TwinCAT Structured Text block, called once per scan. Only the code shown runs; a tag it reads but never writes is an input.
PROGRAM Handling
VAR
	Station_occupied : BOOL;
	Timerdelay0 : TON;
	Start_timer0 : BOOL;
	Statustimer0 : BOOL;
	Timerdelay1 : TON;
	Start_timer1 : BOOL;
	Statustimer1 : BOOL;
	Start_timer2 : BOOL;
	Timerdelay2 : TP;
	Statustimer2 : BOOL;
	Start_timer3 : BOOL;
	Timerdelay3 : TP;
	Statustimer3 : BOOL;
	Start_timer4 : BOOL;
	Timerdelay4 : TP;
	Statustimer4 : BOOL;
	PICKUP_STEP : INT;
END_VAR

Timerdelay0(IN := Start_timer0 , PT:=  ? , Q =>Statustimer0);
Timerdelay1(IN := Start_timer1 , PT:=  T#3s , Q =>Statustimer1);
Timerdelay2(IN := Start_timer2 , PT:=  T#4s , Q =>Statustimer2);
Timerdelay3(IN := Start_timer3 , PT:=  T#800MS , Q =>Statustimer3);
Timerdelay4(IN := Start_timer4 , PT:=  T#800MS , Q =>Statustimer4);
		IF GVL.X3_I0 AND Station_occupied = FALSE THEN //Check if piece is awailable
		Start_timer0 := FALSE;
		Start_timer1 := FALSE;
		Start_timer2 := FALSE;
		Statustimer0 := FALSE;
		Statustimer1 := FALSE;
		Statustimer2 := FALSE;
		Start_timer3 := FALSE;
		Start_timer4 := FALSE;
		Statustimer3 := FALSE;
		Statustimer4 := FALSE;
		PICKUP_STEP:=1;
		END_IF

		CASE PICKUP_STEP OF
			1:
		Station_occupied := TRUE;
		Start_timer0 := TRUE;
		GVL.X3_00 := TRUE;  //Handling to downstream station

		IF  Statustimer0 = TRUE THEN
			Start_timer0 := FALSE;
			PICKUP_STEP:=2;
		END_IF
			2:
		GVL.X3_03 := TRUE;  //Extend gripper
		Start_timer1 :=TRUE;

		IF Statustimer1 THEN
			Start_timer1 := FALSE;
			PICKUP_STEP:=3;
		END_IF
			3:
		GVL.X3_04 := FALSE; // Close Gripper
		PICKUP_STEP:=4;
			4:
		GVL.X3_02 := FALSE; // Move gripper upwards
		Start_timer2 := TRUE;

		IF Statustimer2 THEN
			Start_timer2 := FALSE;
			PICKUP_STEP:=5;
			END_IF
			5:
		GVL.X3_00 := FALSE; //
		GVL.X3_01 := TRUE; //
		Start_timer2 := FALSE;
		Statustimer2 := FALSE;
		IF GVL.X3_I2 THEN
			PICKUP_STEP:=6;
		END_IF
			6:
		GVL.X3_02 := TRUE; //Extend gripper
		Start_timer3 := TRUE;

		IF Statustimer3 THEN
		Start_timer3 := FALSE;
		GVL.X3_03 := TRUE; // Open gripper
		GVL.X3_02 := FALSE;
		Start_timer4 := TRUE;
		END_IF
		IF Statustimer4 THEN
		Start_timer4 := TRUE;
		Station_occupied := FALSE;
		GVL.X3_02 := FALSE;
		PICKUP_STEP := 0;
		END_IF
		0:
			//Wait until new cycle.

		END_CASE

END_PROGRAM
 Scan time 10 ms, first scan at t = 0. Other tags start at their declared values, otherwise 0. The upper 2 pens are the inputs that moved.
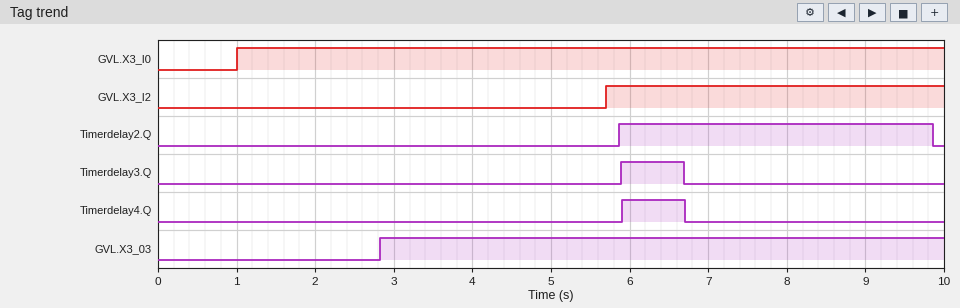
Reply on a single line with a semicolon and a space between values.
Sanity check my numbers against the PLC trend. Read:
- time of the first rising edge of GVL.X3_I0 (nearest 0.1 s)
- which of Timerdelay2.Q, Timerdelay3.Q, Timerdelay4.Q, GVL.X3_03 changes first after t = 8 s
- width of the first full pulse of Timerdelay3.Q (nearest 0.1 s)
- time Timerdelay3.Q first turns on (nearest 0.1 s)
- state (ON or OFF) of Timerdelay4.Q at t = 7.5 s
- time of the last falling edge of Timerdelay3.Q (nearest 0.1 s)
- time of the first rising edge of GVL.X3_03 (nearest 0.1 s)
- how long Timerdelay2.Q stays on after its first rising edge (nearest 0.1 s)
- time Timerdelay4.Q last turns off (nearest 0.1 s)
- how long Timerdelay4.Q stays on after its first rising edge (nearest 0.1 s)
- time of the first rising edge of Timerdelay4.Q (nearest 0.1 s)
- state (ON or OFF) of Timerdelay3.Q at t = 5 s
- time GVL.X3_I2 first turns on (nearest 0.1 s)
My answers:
1.0 s; Timerdelay2.Q; 0.8 s; 5.9 s; OFF; 6.7 s; 2.8 s; 4.0 s; 6.7 s; 0.8 s; 5.9 s; OFF; 5.7 s
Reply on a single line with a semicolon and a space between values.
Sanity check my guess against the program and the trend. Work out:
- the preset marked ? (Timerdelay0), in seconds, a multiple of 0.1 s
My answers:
1.8 s
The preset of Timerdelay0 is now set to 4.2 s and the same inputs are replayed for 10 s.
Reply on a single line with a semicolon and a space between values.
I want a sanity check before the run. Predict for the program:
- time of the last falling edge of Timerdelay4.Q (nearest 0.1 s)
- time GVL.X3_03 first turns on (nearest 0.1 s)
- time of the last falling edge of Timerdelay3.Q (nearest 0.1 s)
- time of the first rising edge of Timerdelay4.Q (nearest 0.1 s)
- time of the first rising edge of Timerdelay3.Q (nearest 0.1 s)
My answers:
9.1 s; 5.2 s; 9.1 s; 8.3 s; 8.3 s
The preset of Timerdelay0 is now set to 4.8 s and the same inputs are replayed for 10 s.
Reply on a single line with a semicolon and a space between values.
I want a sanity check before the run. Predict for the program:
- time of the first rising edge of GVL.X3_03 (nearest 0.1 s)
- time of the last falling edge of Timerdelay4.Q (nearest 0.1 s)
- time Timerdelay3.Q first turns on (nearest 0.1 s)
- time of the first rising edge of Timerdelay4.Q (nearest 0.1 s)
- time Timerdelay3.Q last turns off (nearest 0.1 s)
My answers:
5.8 s; 9.7 s; 8.9 s; 8.9 s; 9.7 s
